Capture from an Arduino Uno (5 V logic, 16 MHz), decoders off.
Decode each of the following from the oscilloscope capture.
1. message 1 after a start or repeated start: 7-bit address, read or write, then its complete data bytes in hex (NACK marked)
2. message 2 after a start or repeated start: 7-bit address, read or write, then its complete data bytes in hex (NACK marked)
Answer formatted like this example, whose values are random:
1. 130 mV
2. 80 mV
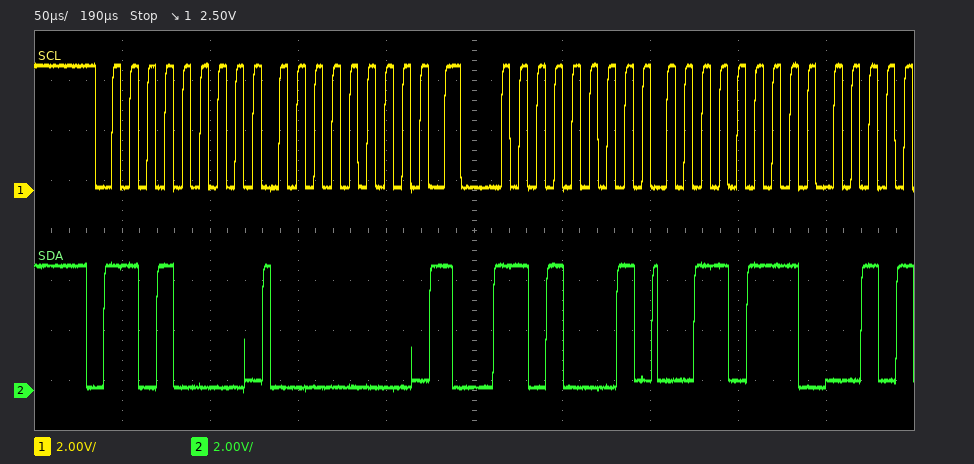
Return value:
1. 0x68 write: 00
2. 0x68 read: 37
